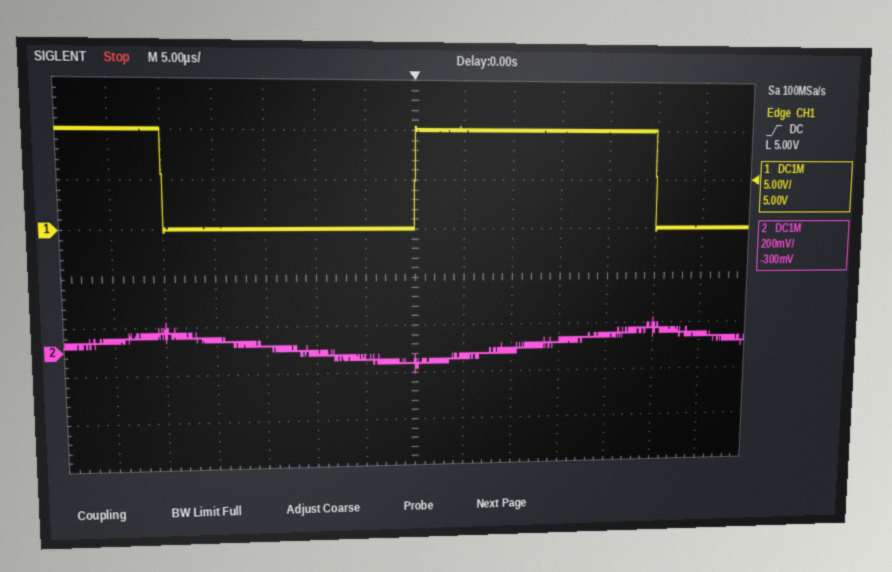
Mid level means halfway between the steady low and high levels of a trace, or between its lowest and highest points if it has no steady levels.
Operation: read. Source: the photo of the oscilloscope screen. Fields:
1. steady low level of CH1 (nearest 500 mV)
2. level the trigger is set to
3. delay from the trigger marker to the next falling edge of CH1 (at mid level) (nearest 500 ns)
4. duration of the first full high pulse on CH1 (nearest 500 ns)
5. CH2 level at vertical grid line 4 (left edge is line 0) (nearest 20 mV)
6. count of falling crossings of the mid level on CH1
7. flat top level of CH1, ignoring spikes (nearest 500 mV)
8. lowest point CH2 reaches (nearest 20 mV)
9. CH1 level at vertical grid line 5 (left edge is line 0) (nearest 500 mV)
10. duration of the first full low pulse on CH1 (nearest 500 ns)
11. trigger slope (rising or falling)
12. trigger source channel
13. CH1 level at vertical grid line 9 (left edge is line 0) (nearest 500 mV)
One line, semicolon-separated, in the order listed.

0.0 V; 5.00 V; 25.0 µs; 25.0 µs; 20 mV; 2; 10.0 V; -100 mV; 0.0 V; 25.0 µs; rising; CH1; 10.0 V
